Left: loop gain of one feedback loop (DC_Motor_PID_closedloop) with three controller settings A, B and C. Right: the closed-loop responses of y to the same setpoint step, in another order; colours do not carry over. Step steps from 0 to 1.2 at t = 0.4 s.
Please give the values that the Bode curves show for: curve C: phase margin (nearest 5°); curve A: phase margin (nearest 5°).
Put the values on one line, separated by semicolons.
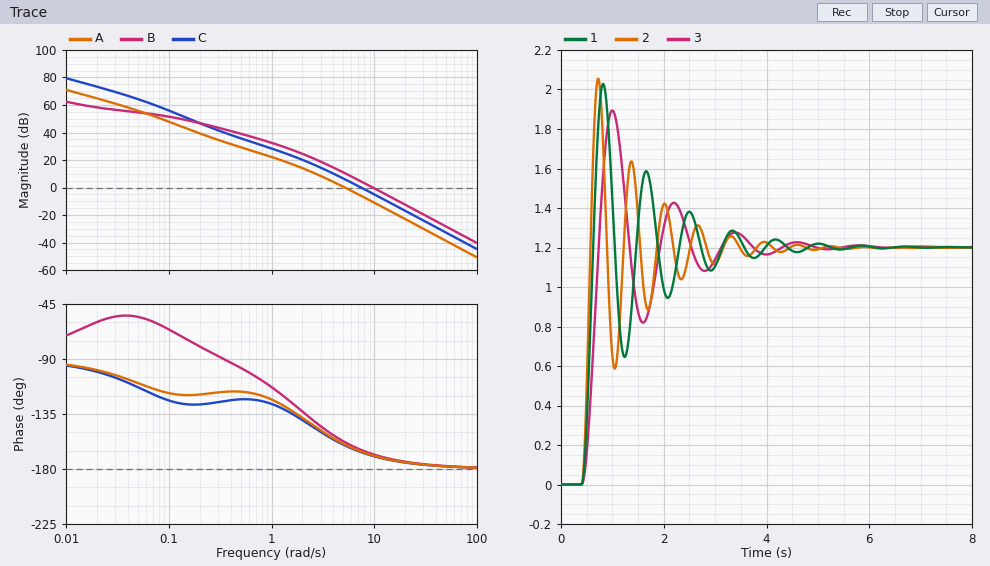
15°; 20°
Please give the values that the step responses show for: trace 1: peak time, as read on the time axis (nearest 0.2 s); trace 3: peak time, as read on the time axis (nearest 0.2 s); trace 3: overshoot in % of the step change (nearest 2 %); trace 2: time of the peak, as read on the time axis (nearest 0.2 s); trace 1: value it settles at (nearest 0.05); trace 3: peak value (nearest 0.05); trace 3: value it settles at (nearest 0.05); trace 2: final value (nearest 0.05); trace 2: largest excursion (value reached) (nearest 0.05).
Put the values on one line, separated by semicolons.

0.8 s; 1.0 s; 58 %; 0.8 s; 1.20; 1.90; 1.20; 1.20; 2.05
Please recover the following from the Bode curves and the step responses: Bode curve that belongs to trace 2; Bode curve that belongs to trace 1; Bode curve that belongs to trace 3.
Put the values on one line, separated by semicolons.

B; C; A
